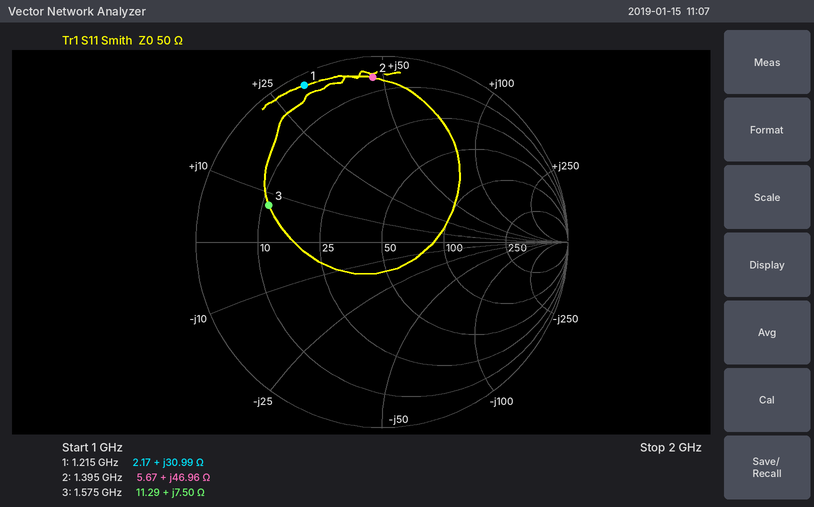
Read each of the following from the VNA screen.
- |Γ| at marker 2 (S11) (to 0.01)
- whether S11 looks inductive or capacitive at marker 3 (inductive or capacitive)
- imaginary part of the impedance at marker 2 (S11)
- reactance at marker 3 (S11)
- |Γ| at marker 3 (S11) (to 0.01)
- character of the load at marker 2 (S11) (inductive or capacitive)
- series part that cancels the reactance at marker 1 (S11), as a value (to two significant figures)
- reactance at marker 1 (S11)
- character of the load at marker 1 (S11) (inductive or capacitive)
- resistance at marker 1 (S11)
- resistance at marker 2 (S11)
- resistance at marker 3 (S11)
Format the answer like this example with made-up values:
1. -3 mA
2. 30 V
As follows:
1. 0.89
2. inductive
3. +46.96 Ω
4. +7.50 Ω
5. 0.64
6. inductive
7. 4.2 pF
8. +30.99 Ω
9. inductive
10. 2.17 Ω
11. 5.67 Ω
12. 11.29 Ω
